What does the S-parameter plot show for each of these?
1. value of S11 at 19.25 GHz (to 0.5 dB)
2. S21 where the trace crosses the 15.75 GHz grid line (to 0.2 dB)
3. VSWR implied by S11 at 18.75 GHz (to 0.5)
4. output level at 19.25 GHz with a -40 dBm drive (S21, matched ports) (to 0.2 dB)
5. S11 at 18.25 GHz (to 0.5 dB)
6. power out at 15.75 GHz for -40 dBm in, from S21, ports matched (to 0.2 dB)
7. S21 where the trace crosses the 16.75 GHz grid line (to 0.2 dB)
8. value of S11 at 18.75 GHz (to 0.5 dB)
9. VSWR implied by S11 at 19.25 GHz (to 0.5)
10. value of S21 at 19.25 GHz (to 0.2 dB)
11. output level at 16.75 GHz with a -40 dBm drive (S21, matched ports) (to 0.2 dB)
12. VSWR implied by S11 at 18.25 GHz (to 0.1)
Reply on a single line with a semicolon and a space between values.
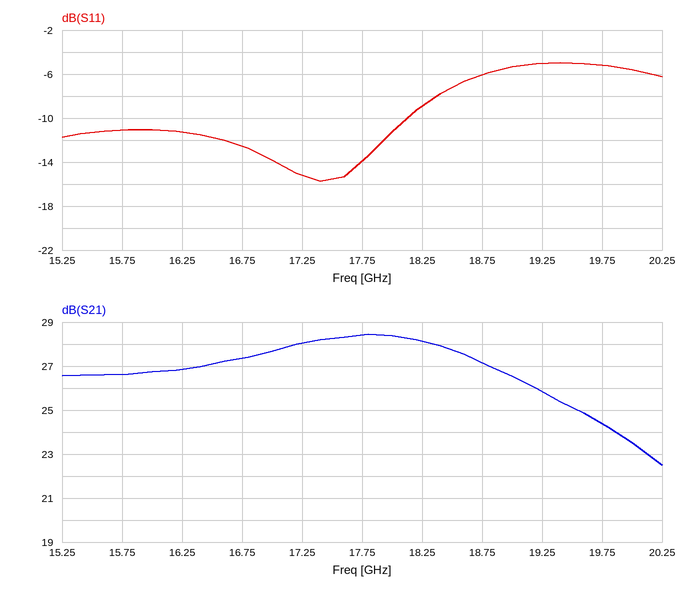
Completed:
-5.0 dB; 26.6 dB; 3.0; -14.2 dBm; -9.0 dB; -13.4 dBm; 27.4 dB; -6.0 dB; 3.5; 25.8 dB; -12.6 dBm; 2.1
